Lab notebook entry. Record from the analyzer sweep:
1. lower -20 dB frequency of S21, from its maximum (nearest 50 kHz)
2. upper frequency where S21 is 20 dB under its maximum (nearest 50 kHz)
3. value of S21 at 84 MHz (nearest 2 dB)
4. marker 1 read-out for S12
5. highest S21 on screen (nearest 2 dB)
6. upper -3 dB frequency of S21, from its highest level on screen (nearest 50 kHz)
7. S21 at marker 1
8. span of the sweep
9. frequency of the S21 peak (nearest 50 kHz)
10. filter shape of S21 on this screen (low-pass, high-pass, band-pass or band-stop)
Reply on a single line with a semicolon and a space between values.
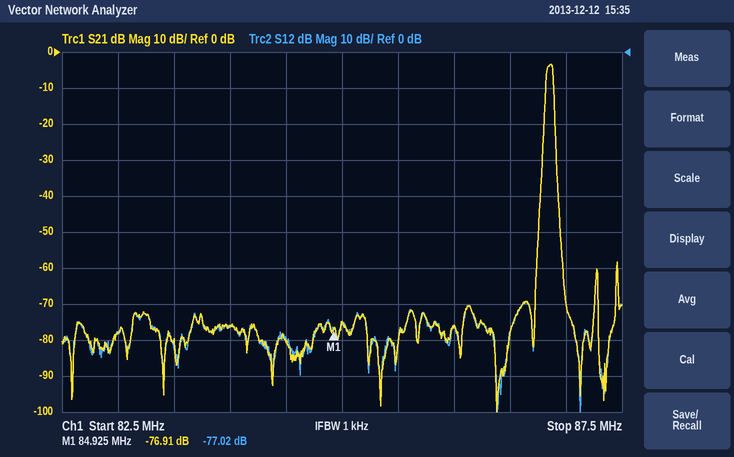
86.80 MHz; 86.90 MHz; -76 dB; -77.02 dB; -4 dB; 86.90 MHz; -76.91 dB; 5 MHz; 86.85 MHz; band-pass
